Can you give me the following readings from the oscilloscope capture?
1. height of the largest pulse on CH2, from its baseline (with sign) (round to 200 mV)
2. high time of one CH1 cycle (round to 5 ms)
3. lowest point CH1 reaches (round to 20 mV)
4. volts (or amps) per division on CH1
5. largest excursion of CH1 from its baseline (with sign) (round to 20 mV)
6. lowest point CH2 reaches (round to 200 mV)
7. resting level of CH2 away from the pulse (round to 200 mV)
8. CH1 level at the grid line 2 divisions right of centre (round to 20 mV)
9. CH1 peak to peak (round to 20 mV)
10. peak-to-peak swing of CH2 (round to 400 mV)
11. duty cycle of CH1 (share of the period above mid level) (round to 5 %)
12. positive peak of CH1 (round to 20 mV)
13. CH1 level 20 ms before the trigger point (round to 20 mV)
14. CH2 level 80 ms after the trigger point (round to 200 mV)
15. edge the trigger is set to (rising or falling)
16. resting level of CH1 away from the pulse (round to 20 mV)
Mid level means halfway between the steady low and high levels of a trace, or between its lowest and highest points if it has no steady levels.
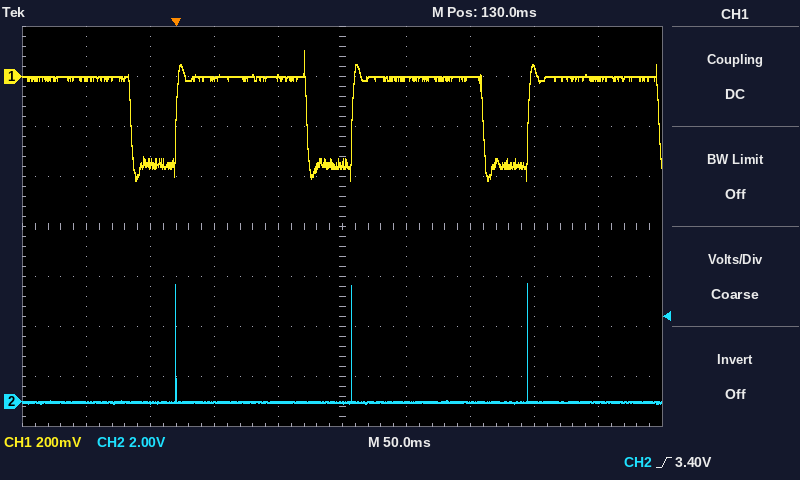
+4.8 V
100 ms
-420 mV
200 mV
-420 mV
0.0 V
0.0 V
0 mV
520 mV
4.8 V
75 %
100 mV
-340 mV
0.0 V
rising
0 mV
